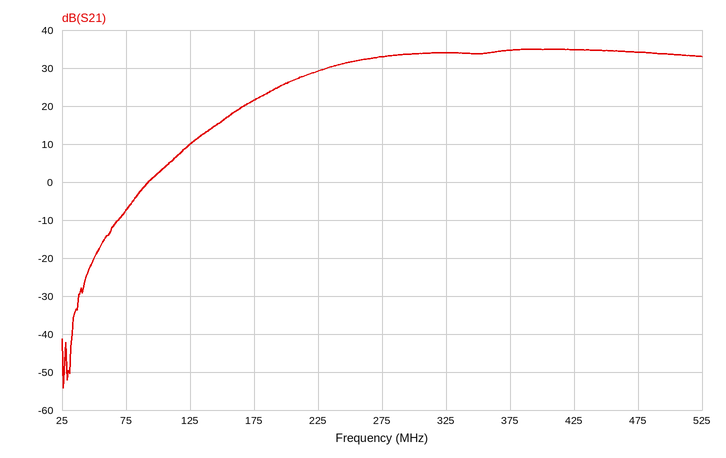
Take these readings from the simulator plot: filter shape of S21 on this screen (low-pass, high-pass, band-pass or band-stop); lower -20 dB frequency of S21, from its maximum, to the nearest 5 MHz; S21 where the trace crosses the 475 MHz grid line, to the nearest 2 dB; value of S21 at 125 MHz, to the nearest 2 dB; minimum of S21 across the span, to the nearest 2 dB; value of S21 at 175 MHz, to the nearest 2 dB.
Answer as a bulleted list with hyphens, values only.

- high-pass
- 145 MHz
- 34 dB
- 10 dB
- -54 dB
- 22 dB
